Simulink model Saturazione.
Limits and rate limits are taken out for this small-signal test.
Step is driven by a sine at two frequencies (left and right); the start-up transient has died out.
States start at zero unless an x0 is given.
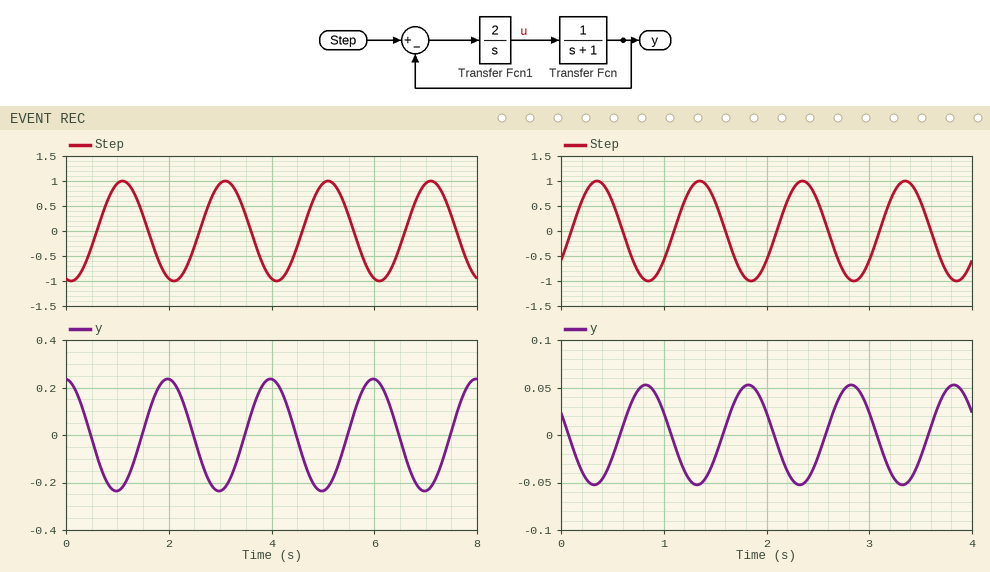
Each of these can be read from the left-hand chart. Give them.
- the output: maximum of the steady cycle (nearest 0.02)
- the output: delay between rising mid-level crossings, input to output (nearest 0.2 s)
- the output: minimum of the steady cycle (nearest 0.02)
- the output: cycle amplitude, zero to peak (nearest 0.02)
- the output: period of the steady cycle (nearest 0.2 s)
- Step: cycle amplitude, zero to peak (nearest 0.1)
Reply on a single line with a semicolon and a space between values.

0.24; 0.8 s; -0.24; 0.24; 2.0 s; 1.0
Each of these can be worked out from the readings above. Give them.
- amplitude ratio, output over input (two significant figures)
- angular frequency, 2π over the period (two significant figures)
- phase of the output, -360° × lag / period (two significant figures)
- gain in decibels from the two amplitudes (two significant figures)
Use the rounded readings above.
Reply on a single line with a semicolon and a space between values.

0.24; 3.1 rad/s; -140°; -12 dB
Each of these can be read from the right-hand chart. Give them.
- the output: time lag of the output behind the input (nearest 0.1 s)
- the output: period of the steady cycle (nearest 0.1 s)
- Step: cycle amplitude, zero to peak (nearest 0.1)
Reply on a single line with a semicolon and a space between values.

0.5 s; 1.0 s; 1.0
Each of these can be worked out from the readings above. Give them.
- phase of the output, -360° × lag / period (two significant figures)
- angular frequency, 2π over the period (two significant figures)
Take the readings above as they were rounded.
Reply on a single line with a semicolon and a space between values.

-180°; 6.3 rad/s
